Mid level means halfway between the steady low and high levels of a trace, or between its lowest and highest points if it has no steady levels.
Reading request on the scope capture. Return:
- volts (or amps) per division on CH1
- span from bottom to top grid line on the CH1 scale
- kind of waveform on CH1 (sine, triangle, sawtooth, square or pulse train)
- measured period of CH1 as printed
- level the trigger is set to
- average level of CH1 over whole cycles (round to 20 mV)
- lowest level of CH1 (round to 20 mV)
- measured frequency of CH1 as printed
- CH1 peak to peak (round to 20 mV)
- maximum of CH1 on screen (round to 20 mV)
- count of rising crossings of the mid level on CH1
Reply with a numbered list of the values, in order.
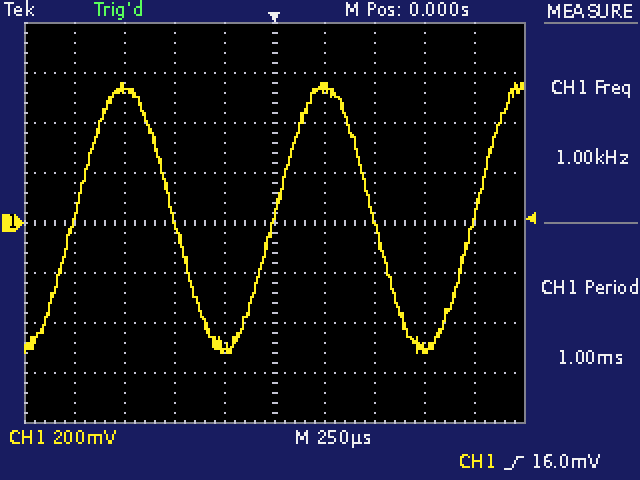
1. 200 mV
2. 1.6 V
3. sine
4. 1.00 ms
5. 16.0 mV
6. 20 mV
7. -520 mV
8. 1.00 kHz
9. 1.08 V
10. 560 mV
11. 3
